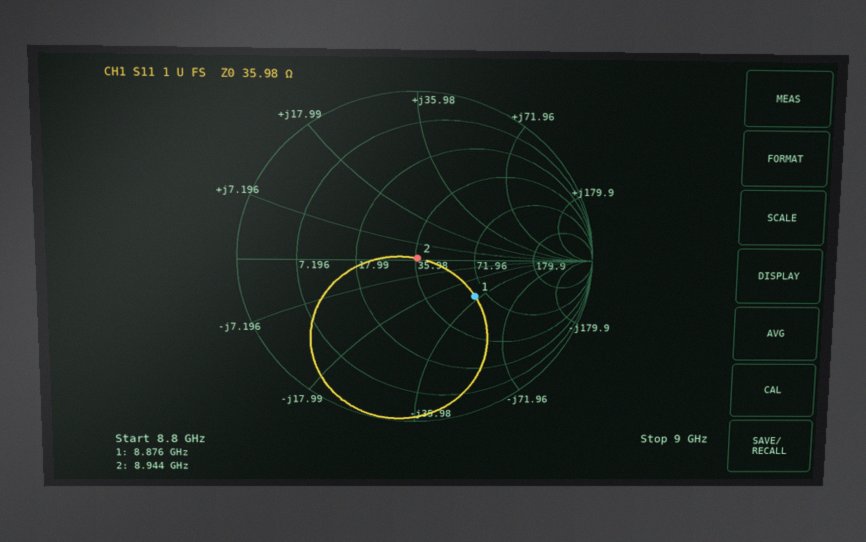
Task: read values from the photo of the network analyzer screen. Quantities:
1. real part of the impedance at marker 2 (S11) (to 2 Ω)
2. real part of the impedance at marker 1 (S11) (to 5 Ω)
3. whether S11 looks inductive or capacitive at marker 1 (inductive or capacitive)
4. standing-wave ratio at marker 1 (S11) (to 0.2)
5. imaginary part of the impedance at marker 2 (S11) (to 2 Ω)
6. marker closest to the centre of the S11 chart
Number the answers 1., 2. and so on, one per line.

1. 36 Ω
2. 60 Ω
3. capacitive
4. 2.4
5. 0 Ω
6. marker 2
